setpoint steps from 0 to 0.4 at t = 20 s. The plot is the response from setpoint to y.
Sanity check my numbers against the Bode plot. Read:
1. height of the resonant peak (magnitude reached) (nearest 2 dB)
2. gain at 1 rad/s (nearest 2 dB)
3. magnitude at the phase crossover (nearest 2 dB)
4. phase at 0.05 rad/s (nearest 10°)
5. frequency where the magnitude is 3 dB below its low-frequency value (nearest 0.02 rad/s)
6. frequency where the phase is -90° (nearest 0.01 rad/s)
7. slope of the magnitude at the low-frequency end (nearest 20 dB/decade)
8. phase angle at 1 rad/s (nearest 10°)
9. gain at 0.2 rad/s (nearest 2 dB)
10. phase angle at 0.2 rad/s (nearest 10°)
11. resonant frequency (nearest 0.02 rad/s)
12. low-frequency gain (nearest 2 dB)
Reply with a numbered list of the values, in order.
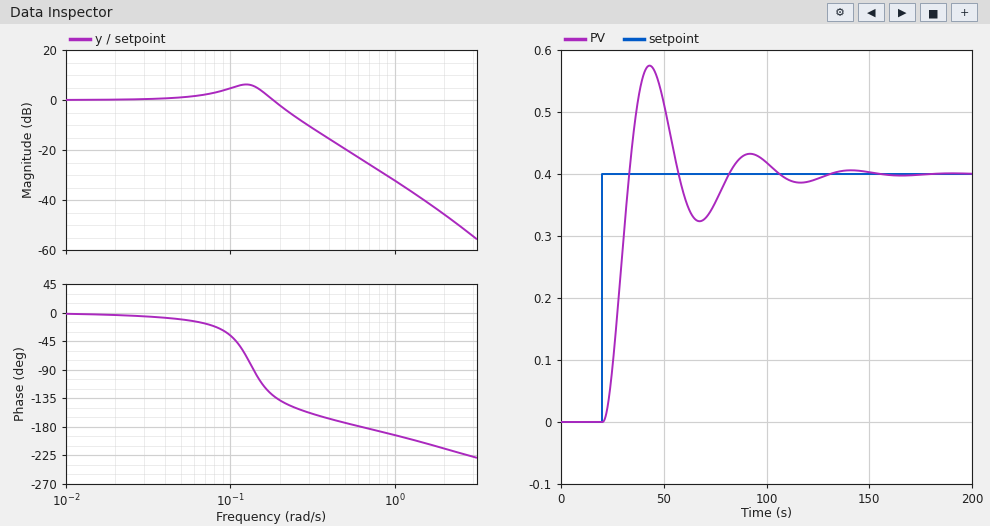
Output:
1. 6 dB
2. -32 dB
3. -24 dB
4. -10°
5. 0.20 rad/s
6. 0.14 rad/s
7. 0 dB/decade
8. -190°
9. -2 dB
10. -140°
11. 0.12 rad/s
12. 0 dB
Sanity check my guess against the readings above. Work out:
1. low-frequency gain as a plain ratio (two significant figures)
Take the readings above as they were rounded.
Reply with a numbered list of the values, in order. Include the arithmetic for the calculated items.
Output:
1. 10^(0 / 20) = 1.0
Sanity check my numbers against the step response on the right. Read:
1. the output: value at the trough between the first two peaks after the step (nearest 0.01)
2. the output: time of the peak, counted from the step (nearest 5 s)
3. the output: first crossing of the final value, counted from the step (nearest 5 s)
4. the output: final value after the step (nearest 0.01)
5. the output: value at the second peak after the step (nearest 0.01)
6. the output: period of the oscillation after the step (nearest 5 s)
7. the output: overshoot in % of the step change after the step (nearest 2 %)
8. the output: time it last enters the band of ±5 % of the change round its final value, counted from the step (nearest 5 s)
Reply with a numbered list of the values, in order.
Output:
1. 0.32
2. 25 s
3. 15 s
4. 0.40
5. 0.43
6. 50 s
7. 44 %
8. 80 s
